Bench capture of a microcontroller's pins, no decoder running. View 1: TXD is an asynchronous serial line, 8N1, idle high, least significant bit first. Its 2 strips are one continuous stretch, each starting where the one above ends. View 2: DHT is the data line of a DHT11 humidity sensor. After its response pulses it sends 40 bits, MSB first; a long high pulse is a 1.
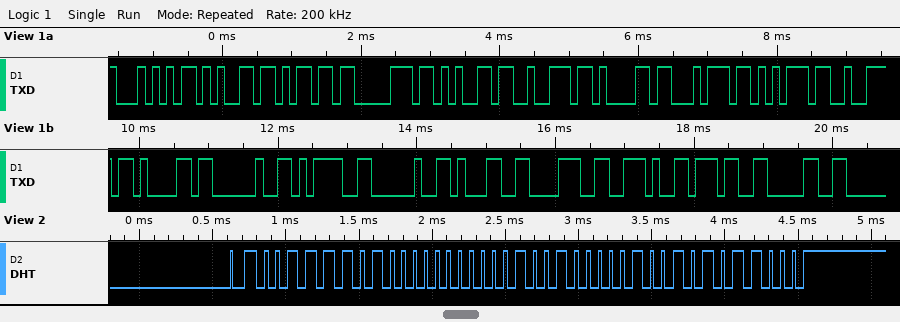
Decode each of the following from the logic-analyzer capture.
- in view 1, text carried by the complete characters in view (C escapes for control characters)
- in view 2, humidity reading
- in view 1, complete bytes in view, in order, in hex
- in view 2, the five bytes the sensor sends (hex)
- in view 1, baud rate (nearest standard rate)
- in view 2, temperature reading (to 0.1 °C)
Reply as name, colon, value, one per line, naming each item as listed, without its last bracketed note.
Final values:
in view 1, text carried by the complete characters in view: "Temperatura = 18.70"
in view 2, humidity reading: 61 %
in view 1, complete bytes in view, in order, in hex: 54 65 6D 70 65 72 61 74 75 72 61 20 3D 20 31 38 2E 37 30
in view 2, the five bytes the sensor sends: 3D 00 12 09 58
in view 1, baud rate: 9600 baud
in view 2, temperature reading: 18.9 °C
